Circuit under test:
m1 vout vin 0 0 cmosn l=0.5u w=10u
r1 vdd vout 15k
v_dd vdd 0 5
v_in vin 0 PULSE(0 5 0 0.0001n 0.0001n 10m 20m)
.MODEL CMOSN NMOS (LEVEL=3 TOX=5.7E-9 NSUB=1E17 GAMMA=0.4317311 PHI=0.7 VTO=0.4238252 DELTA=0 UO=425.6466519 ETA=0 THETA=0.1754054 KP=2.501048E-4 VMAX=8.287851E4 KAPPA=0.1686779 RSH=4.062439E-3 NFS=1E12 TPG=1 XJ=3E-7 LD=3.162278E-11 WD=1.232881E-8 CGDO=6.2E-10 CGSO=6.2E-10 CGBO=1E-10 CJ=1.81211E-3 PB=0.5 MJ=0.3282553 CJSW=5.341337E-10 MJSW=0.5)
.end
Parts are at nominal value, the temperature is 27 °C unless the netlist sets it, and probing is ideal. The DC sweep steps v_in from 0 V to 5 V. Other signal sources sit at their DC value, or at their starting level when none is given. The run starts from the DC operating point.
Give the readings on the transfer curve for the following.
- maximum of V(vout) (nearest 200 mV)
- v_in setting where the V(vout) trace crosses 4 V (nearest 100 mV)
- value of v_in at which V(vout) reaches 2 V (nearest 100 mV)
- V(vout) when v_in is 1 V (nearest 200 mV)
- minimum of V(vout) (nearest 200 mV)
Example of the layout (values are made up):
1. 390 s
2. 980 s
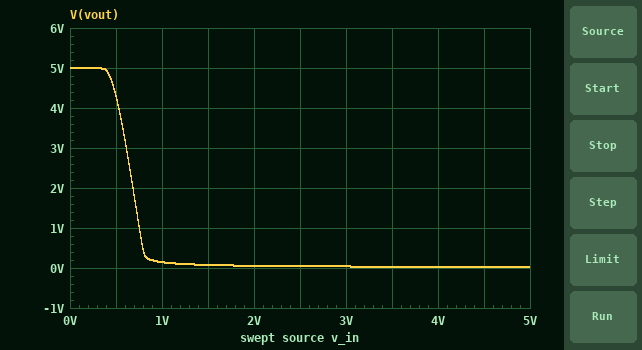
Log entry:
1. 5.0 V
2. 500 mV
3. 700 mV
4. 200 mV
5. 0 V
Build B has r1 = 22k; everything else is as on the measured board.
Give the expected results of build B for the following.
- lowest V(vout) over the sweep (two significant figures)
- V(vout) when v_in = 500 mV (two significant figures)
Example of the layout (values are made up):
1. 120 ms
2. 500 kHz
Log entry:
1. 18 mV
2. 4.0 V
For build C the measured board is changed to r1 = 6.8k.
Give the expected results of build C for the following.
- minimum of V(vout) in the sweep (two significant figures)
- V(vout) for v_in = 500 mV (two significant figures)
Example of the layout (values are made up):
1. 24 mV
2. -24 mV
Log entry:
1. 59 mV
2. 4.7 V
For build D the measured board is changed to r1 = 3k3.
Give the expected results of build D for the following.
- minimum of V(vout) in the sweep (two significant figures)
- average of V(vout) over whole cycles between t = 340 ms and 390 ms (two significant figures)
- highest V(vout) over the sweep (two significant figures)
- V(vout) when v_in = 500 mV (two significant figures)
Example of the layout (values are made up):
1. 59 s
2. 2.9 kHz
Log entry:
1. 130 mV
2. 2.6 V
3. 5.0 V
4. 4.8 V
